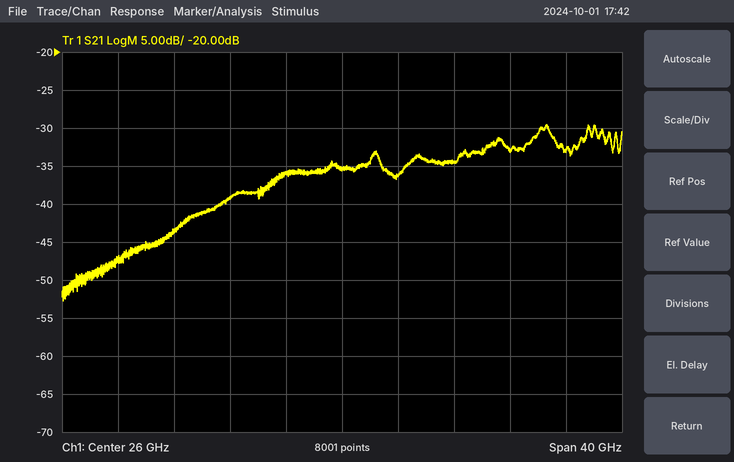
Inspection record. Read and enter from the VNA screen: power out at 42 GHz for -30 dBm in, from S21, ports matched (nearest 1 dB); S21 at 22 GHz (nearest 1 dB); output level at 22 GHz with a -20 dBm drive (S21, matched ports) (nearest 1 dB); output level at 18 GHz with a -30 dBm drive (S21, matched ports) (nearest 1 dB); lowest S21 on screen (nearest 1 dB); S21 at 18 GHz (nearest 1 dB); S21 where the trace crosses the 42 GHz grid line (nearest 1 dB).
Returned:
-63 dBm
-36 dB
-56 dBm
-69 dBm
-53 dB
-39 dB
-33 dB
